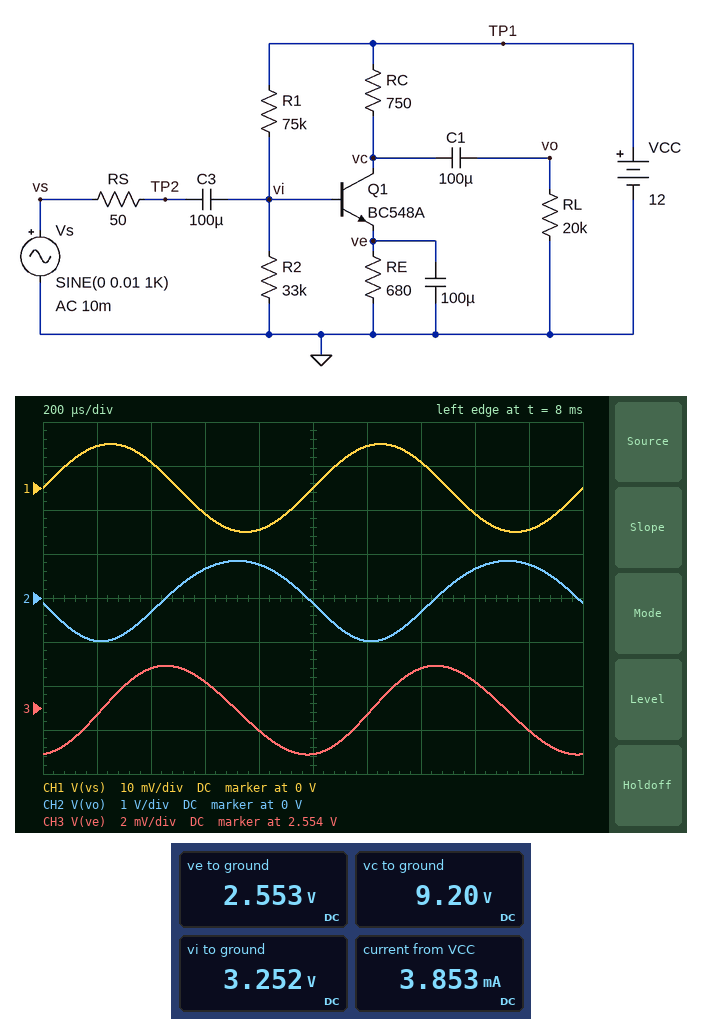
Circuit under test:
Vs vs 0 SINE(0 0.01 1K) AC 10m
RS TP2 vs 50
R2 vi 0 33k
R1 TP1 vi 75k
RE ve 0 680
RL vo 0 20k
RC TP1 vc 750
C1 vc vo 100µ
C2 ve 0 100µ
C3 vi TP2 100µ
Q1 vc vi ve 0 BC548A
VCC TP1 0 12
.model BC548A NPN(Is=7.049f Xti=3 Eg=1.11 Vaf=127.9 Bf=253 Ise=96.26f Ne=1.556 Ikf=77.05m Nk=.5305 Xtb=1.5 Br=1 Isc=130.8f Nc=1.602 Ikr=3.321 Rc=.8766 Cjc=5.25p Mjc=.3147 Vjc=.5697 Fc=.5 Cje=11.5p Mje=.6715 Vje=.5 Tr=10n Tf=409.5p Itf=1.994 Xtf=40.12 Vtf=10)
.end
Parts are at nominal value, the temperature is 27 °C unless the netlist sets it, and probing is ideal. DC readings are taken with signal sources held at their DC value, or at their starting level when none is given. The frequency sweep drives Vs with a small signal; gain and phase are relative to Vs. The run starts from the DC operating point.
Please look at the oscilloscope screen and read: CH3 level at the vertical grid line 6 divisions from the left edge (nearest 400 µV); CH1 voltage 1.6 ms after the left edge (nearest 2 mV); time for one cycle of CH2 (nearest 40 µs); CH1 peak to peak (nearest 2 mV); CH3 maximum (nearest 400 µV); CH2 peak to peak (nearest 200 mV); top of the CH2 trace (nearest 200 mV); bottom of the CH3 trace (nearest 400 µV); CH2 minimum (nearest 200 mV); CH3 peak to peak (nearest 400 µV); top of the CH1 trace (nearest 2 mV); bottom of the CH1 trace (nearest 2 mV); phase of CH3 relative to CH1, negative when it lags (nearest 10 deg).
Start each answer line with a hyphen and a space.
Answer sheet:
- 2.5536 V
- -6 mV
- 1.00 ms
- 20 mV
- 2.5560 V
- 1.8 V
- 800 mV
- 2.5520 V
- -1.0 V
- 4.0 mV
- 10 mV
- -10 mV
- -80 deg
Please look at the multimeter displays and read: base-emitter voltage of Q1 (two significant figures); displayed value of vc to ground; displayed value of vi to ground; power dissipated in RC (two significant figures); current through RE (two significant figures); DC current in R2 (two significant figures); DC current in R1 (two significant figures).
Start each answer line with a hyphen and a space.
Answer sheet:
- 700 mV
- 9.20 V
- 3.252 V
- 10 mW
- 3.8 mA
- 99 µA
- 120 µA
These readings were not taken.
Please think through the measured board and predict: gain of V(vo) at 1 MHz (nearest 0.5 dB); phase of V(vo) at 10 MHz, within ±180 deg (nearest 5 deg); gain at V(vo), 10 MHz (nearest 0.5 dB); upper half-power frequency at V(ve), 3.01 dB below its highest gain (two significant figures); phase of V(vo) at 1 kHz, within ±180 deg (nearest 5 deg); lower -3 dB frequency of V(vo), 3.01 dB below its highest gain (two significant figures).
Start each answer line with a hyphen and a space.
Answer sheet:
- 39.5 dB
- 130 deg
- 36.0 dB
- 210 Hz
- -170 deg
- 210 Hz
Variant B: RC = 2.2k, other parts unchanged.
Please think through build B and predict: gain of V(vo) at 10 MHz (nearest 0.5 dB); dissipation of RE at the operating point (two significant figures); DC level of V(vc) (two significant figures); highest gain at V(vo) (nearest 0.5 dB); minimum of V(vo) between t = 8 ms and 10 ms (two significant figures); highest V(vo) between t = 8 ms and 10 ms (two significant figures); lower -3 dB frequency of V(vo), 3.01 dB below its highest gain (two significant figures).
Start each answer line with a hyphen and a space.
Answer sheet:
- 35.5 dB
- 9.5 mW
- 3.8 V
- 48.0 dB
- -1.2 V
- 2.0 V
- 200 Hz
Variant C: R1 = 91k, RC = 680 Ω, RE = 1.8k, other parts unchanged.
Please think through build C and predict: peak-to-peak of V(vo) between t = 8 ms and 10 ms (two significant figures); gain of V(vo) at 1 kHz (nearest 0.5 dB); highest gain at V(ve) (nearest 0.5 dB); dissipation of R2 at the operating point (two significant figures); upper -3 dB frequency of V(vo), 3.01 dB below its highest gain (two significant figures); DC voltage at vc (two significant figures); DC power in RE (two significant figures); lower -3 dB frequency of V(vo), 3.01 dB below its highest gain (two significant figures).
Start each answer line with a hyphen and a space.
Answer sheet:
- 630 mV
- 30.0 dB
- 0 dB
- 280 µW
- 21 MHz
- 11 V
- 3.1 mW
- 79 Hz
